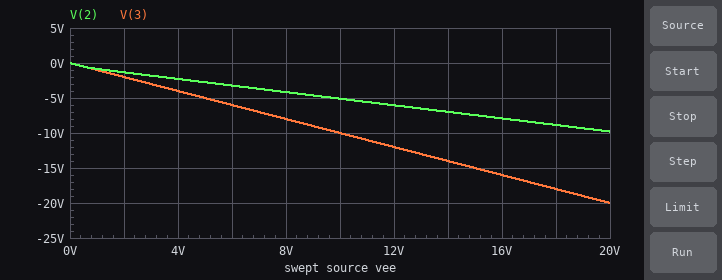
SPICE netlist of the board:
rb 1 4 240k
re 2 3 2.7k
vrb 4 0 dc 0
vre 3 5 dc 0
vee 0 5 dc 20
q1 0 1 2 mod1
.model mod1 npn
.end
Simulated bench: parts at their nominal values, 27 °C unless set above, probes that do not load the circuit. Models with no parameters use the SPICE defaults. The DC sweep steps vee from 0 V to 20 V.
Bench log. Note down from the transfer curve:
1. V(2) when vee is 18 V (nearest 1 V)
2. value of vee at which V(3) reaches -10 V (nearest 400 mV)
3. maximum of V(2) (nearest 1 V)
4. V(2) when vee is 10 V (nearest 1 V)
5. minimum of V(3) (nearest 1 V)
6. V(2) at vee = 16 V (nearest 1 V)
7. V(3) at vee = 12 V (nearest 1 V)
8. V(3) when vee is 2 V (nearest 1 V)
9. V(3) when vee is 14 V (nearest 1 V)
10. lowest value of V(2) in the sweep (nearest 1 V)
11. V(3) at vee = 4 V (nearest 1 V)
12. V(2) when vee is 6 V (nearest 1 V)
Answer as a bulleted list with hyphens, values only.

- -9 V
- 10.0 V
- 0 V
- -5 V
- -20 V
- -8 V
- -12 V
- -2 V
- -14 V
- -10 V
- -4 V
- -3 V
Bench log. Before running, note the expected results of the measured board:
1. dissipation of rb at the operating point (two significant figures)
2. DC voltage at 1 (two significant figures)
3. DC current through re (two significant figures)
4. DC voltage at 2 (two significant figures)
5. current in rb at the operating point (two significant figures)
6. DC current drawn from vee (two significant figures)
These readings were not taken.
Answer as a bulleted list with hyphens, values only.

- 340 µW
- -9.0 V
- 3.8 mA
- -9.8 V
- 37 µA
- 3.8 mA
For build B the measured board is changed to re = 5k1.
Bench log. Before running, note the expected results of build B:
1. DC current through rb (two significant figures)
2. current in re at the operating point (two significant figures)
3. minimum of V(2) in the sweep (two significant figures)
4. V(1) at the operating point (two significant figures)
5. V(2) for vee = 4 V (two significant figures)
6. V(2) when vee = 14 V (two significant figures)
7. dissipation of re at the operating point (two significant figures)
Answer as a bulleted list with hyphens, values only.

- 25 µA
- 2.6 mA
- -6.9 V
- -6.1 V
- -1.8 V
- -5.0 V
- 34 mW
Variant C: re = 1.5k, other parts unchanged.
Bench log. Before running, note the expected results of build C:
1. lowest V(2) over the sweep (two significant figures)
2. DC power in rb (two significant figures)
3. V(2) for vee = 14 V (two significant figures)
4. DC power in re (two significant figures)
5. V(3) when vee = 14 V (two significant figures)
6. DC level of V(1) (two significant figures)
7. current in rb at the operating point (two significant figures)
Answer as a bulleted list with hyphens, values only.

- -13 V
- 580 µW
- -8.9 V
- 37 mW
- -14 V
- -12 V
- 49 µA
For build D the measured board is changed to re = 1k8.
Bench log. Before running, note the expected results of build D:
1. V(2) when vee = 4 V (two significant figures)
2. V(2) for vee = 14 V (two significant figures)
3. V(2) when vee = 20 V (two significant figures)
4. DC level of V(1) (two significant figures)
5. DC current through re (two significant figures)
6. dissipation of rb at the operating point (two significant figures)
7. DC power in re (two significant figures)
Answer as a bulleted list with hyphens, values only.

- -2.6 V
- -8.3 V
- -12 V
- -11 V
- 4.6 mA
- 500 µW
- 38 mW
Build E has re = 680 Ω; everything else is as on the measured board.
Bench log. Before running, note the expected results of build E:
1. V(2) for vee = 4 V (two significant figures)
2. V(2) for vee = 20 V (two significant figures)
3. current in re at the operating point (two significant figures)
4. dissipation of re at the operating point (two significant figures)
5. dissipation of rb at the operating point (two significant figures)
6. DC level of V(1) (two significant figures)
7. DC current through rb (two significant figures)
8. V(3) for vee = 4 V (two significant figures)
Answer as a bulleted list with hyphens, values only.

- -3.3 V
- -16 V
- 6.3 mA
- 27 mW
- 930 µW
- -15 V
- 62 µA
- -4.0 V
